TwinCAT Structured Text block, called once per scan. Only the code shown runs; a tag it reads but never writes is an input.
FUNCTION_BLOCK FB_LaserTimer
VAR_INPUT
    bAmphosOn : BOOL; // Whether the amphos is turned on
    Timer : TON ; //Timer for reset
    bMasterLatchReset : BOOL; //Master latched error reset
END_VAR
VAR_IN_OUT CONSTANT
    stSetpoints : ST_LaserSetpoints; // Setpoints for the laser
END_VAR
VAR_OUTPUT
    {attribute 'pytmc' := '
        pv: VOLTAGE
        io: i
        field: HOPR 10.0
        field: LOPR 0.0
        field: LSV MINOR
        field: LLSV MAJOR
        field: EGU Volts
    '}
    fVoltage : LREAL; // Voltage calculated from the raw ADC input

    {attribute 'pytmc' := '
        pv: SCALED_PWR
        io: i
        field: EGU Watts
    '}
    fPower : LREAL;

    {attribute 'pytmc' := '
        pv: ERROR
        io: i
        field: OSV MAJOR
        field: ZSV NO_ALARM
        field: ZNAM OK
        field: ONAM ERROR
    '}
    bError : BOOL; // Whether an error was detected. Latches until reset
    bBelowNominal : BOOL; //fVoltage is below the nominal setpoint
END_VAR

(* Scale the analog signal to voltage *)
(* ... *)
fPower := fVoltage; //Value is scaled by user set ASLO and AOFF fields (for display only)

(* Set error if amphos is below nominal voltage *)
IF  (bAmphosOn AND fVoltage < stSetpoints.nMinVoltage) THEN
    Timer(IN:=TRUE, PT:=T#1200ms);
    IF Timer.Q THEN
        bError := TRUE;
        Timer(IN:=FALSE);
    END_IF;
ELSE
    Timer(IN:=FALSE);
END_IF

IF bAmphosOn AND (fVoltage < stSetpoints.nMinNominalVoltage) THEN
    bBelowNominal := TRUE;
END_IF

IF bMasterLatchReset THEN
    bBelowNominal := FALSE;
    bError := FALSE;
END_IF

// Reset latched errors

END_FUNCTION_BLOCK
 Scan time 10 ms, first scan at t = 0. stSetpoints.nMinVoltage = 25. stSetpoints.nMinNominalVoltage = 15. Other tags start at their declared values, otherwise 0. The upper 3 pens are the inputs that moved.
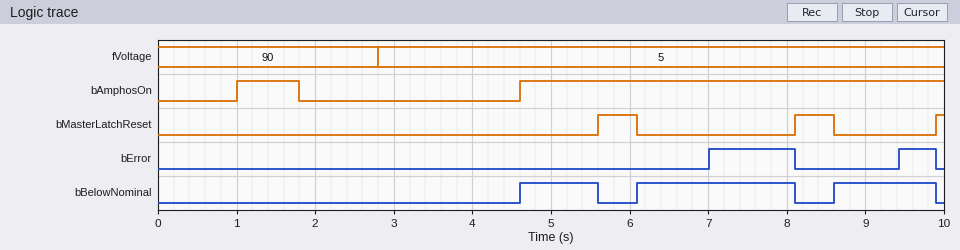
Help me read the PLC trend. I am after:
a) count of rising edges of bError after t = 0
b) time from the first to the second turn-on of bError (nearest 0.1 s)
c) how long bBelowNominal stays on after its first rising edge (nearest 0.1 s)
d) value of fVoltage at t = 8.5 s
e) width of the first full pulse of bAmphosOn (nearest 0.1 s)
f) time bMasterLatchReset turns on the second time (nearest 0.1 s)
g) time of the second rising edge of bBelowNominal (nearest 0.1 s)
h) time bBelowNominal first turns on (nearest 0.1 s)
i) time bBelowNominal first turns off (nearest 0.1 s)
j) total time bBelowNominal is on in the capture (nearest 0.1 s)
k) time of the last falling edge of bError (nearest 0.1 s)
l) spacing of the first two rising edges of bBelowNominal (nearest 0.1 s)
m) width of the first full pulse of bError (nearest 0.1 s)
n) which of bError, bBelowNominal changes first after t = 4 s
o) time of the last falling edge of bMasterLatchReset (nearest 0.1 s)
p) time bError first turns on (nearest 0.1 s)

2
2.4 s
1.0 s
5
0.8 s
8.1 s
6.1 s
4.6 s
5.6 s
4.3 s
9.9 s
1.5 s
1.1 s
bBelowNominal
8.6 s
7.0 s
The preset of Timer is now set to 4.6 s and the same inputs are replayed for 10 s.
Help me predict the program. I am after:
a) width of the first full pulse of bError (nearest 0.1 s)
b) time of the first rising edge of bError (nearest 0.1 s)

0.7 s
9.2 s
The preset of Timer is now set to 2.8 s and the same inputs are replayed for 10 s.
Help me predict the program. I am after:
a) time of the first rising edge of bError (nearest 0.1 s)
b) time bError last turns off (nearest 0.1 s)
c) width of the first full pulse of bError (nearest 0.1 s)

7.4 s
8.1 s
0.7 s
